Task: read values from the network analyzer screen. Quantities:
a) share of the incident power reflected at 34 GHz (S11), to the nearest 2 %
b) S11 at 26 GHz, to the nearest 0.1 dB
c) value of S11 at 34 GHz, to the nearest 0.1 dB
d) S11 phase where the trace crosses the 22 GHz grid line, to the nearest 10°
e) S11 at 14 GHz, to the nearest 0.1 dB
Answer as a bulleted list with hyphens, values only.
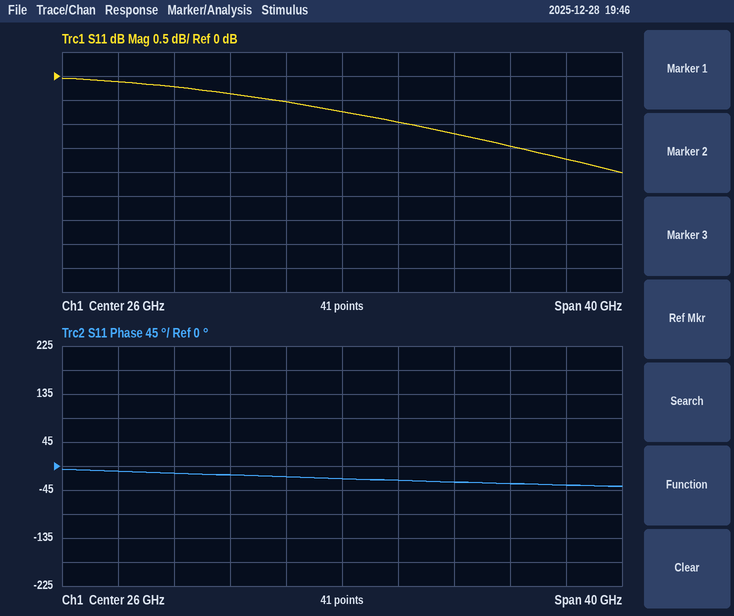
- 76 %
- -0.7 dB
- -1.2 dB
- -20°
- -0.2 dB
